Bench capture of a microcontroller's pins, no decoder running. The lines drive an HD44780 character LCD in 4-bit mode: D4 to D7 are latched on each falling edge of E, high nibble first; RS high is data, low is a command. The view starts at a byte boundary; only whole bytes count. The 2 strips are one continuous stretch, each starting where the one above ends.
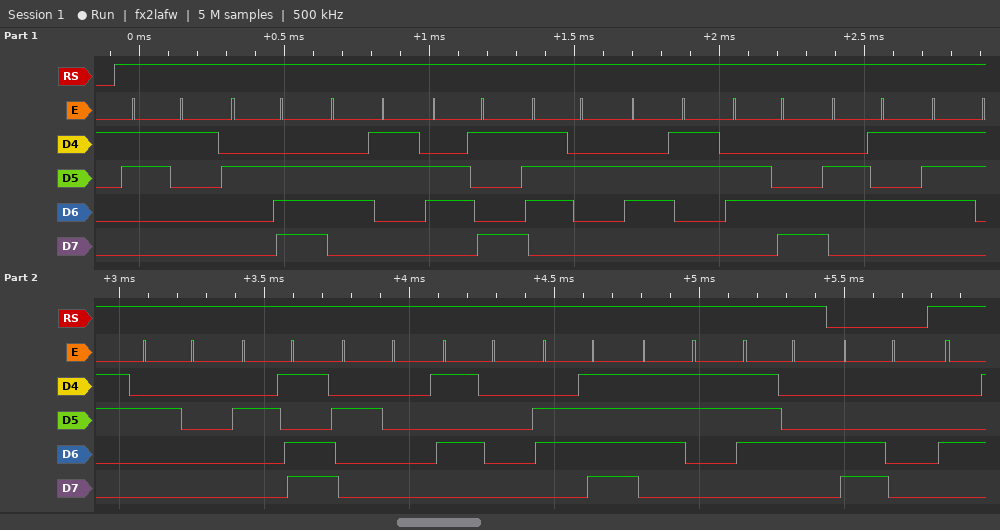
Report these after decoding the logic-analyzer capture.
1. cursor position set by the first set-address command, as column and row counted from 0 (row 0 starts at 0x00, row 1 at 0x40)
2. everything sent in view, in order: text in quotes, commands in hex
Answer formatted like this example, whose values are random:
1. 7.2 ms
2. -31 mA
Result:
1. column 0, row 1
2. "1.circles - Post" 0xC0
